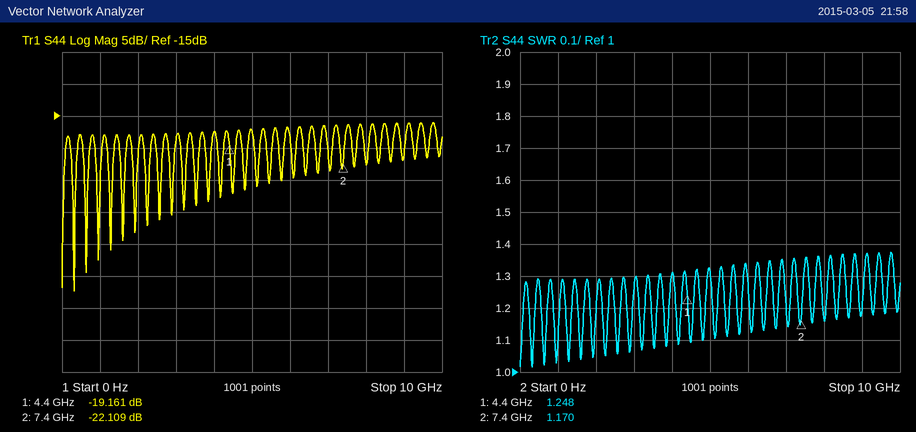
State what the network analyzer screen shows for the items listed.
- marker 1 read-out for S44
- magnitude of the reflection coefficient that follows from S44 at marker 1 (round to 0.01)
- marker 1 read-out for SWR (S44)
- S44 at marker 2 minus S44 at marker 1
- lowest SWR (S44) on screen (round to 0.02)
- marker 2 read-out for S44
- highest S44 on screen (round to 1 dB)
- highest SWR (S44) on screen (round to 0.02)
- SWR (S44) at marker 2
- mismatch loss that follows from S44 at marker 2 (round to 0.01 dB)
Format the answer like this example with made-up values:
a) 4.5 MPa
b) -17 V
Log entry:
a) -19.161 dB
b) 0.11
c) 1.248
d) -2.948 dB
e) 1.02
f) -22.109 dB
g) -16 dB
h) 1.38
i) 1.170
j) 0.03 dB
